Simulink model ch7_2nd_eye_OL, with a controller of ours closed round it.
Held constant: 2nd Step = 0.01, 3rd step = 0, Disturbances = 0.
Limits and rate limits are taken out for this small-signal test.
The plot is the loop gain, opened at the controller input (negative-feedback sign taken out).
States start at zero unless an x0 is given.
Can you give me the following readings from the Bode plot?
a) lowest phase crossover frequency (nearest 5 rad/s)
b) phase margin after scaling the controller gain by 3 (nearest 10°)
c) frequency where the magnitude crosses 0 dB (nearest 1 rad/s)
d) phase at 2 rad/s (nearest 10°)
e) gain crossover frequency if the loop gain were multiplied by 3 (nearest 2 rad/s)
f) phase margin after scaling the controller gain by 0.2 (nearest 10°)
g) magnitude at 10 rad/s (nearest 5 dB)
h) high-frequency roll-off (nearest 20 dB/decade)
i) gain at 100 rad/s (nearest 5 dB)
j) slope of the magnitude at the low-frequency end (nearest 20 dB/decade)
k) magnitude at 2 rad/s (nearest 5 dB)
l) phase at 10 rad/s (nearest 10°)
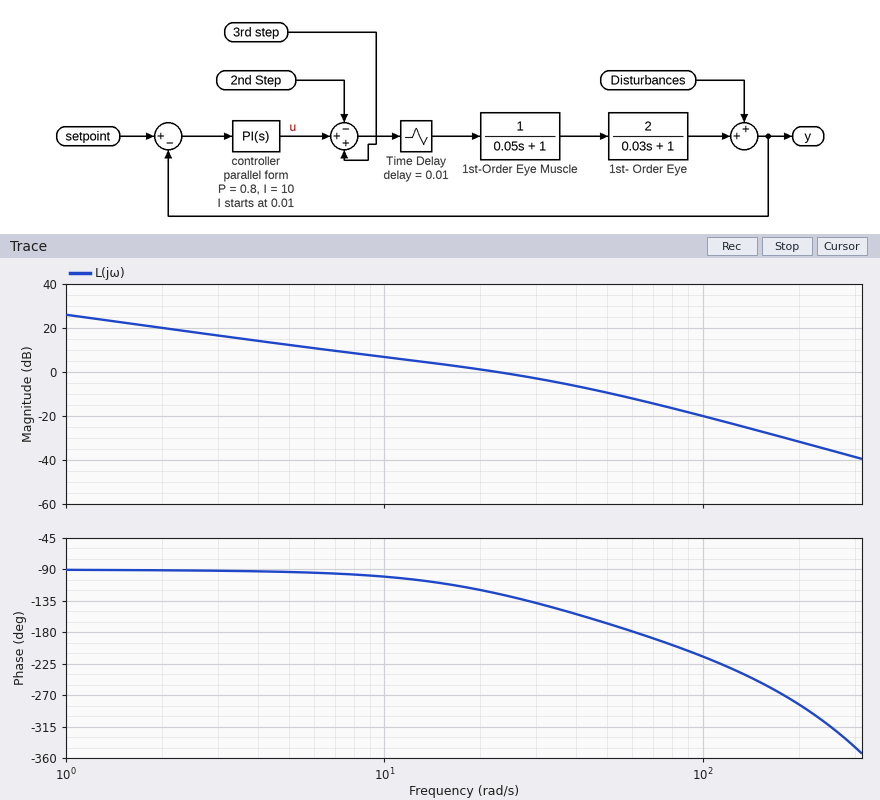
60 rad/s
10°
23 rad/s
-90°
50 rad/s
90°
5 dB
-40 dB/decade
-20 dB
-20 dB/decade
20 dB
-100°
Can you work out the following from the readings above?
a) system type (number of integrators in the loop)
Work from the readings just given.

1
